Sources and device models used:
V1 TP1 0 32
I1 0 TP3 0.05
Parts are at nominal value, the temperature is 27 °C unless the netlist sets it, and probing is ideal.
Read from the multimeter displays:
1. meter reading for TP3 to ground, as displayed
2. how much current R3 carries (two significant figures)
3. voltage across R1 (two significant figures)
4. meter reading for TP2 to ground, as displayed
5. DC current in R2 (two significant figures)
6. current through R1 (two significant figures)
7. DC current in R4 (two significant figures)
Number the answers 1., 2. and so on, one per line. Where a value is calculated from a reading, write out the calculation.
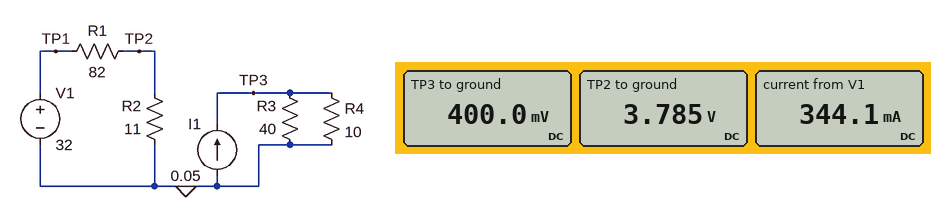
1. 400.0 mV
2. (400 mV) / 40 Ω = 10 mA
3. 32 V - 3.785 V = 28 V
4. 3.785 V
5. (3.785 V) / 11 Ω = 340 mA
6. (32 V - 3.785 V) / 82 Ω = 340 mA
7. (400 mV) / 10 Ω = 40 mA
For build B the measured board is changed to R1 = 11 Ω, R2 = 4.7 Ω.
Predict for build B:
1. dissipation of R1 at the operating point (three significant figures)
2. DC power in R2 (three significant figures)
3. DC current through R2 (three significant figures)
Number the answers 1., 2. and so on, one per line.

1. 45.7 W
2. 19.5 W
3. 2.04 A
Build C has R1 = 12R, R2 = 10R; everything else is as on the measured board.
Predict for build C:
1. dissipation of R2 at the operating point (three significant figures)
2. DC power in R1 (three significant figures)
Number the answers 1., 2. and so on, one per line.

1. 21.2 W
2. 25.4 W
